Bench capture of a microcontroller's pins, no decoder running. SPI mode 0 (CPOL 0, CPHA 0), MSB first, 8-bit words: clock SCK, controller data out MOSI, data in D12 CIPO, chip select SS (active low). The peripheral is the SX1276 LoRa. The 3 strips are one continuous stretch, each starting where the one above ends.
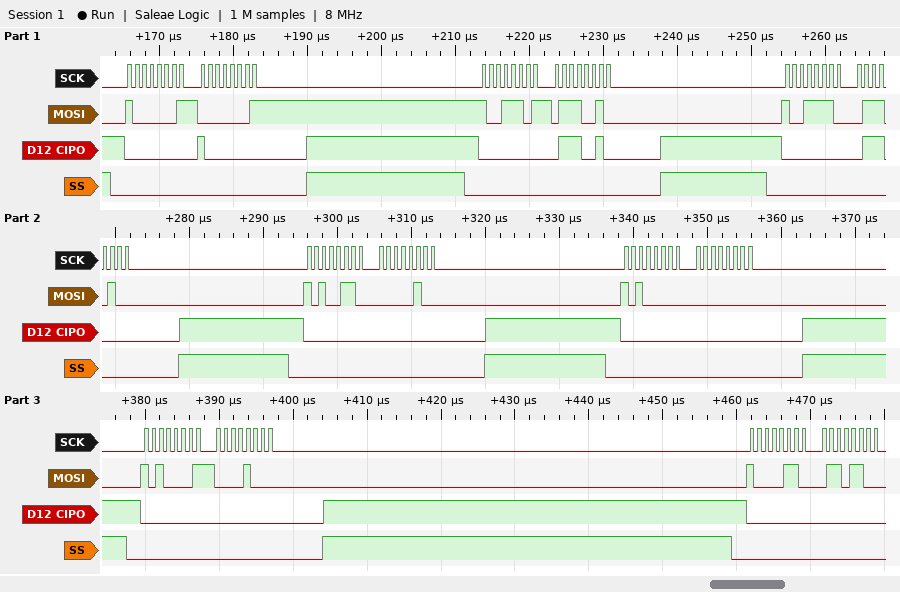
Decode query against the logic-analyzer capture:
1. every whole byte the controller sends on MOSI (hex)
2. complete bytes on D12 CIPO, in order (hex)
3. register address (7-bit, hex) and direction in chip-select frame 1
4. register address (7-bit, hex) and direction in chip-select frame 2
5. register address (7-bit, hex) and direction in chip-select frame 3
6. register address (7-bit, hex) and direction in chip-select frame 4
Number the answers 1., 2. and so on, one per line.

1. 0x81 0x01 0x9D 0x72 0x9E 0x74 0xA6 0x04 0xA0 0x00 0xA1 0x08 0x86 0x6C
2. 0x00 0x80 0x00 0x72 0x00 0x70 0x00 0x00 0x00 0x00 0x00 0x00 0x00 0x00
3. 0x01 write
4. 0x1D write
5. 0x1E write
6. 0x26 write
